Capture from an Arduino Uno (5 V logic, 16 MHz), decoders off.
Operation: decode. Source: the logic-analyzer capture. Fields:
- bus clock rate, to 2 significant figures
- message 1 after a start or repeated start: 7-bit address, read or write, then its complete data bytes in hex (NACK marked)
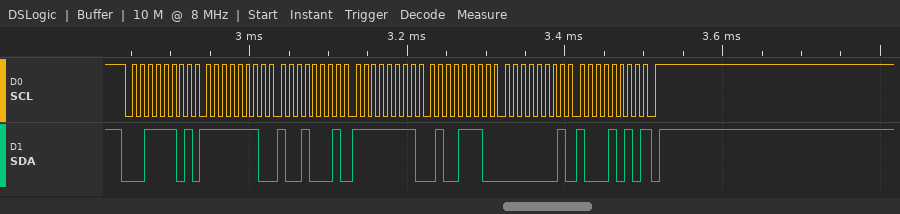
100 kHz
0x1E read: FE 91 FF 4E 01 8A NACK
